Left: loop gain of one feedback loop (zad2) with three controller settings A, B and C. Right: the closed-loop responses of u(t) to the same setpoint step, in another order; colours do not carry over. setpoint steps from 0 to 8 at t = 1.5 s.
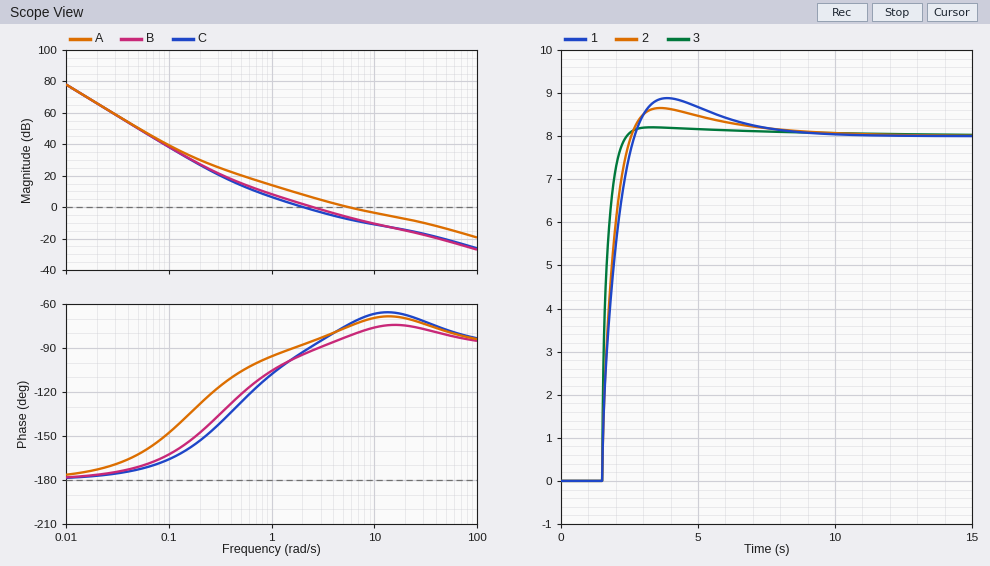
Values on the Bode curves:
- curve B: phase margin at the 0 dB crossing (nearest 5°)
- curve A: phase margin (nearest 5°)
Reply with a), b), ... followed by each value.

a) 90°
b) 105°
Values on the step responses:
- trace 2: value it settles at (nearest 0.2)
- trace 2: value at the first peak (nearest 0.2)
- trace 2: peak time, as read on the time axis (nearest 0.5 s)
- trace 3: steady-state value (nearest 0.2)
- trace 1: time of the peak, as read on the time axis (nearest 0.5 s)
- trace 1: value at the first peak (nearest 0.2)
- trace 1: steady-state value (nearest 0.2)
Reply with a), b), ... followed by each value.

a) 8.0
b) 8.6
c) 3.5 s
d) 8.0
e) 4.0 s
f) 8.8
g) 8.0
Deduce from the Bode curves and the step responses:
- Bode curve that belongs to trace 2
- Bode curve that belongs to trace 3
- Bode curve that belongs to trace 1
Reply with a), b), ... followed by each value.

a) B
b) A
c) C
